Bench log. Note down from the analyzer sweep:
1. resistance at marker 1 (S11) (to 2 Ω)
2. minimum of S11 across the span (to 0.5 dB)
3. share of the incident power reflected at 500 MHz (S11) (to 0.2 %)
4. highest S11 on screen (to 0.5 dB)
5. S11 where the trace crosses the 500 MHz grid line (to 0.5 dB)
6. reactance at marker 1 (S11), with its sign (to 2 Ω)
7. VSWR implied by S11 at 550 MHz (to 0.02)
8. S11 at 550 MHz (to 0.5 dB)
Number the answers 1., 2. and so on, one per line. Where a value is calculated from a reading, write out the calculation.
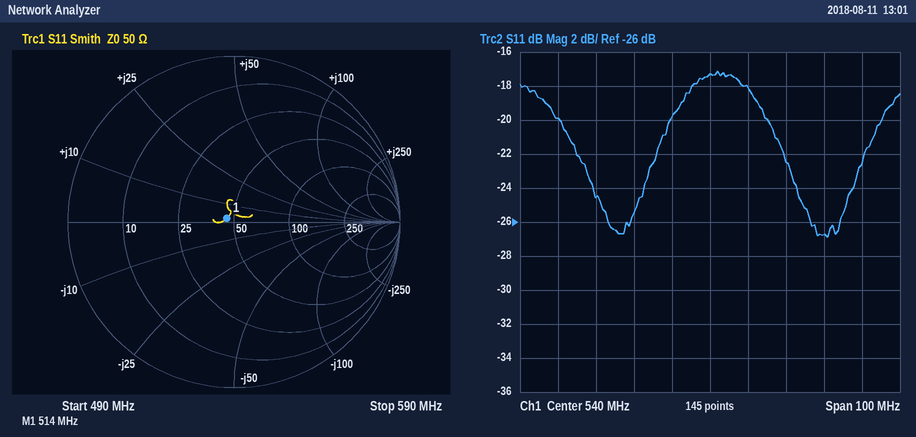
1. 46 Ω
2. -27.0 dB
3. 10^(-20/10) ≈ 1.0 %
4. -17.0 dB
5. -20.0 dB
6. +2 Ω
7. |Γ| = 10^(-18/20) = 0.1259; VSWR = (1 + 0.1259)/(1 − 0.1259) ≈ 1.29, so 1.28 to the nearest 0.02
8. -18.0 dB
